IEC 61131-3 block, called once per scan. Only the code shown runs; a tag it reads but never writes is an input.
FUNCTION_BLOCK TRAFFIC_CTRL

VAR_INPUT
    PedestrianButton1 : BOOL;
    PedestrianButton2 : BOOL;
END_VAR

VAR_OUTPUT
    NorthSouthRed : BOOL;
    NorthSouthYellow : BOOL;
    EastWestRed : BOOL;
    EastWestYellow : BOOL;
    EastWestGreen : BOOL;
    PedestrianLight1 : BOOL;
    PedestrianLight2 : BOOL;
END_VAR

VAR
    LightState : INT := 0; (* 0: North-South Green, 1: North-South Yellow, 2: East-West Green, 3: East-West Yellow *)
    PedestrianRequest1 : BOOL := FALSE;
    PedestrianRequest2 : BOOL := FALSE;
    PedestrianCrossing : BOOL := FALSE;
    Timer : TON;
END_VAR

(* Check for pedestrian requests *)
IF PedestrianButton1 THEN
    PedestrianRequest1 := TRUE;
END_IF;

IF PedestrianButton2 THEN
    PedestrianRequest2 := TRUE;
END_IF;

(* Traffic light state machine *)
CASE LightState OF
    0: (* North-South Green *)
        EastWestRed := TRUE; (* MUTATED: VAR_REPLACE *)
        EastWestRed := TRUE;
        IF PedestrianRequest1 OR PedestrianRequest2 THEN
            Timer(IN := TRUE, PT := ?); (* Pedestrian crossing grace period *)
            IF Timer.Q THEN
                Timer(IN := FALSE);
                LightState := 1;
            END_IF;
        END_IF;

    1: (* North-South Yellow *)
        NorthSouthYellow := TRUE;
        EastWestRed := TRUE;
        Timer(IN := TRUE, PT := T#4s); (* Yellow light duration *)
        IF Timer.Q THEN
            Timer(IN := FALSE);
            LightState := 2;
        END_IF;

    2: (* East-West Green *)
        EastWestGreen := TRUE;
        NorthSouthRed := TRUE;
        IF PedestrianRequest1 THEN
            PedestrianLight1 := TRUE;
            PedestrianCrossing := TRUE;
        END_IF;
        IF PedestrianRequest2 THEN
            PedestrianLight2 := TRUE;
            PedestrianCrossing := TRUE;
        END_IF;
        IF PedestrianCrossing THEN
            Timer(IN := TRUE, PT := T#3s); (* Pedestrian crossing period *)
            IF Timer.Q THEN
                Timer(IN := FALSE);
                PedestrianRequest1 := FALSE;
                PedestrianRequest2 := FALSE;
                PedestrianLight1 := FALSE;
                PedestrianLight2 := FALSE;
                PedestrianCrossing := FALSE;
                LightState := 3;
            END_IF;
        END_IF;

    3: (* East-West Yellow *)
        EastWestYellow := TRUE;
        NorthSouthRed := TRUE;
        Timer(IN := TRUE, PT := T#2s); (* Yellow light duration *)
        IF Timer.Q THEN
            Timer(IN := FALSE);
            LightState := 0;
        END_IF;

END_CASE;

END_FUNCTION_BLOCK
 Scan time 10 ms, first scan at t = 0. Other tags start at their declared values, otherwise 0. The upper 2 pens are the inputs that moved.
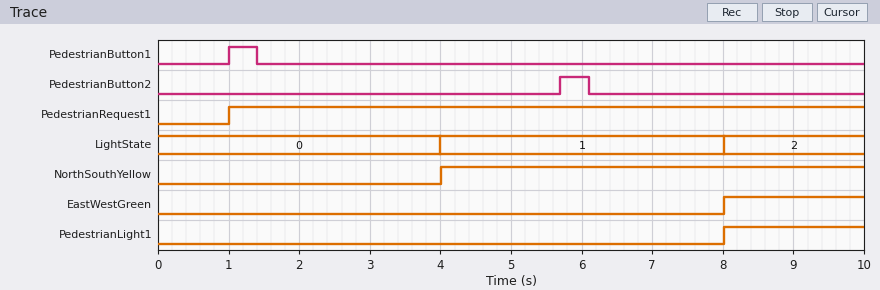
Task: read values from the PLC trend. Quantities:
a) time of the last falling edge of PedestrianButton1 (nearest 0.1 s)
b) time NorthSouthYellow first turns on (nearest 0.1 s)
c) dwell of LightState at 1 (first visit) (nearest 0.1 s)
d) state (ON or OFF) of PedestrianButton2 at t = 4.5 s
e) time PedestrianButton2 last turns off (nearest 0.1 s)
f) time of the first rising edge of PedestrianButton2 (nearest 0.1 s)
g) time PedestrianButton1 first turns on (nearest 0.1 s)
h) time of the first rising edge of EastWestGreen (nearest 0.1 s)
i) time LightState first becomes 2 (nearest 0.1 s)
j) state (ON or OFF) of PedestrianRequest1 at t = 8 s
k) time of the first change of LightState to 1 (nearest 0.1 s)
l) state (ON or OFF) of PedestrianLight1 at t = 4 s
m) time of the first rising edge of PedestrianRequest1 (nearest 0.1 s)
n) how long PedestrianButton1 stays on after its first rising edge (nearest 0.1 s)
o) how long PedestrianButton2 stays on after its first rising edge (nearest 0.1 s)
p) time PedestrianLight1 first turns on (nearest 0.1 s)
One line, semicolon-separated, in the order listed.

1.4 s; 4.0 s; 4.0 s; OFF; 6.1 s; 5.7 s; 1.0 s; 8.0 s; 8.0 s; ON; 4.0 s; OFF; 1.0 s; 0.4 s; 0.4 s; 8.0 s
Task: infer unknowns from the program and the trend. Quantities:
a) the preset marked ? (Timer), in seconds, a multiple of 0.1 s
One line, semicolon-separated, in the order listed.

3.0 s
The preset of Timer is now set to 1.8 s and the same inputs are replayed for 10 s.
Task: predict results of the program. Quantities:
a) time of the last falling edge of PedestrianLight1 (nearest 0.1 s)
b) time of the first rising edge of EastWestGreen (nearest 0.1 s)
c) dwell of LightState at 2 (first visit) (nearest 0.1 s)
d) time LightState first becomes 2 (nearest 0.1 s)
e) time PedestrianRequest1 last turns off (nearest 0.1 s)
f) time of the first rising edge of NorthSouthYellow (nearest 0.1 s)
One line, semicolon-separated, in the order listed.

9.8 s; 6.8 s; 3.0 s; 6.8 s; 9.8 s; 2.8 s
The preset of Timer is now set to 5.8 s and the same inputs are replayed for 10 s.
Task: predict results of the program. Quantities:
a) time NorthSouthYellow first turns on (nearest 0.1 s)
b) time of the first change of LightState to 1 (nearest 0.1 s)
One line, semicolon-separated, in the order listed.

6.8 s; 6.8 s
